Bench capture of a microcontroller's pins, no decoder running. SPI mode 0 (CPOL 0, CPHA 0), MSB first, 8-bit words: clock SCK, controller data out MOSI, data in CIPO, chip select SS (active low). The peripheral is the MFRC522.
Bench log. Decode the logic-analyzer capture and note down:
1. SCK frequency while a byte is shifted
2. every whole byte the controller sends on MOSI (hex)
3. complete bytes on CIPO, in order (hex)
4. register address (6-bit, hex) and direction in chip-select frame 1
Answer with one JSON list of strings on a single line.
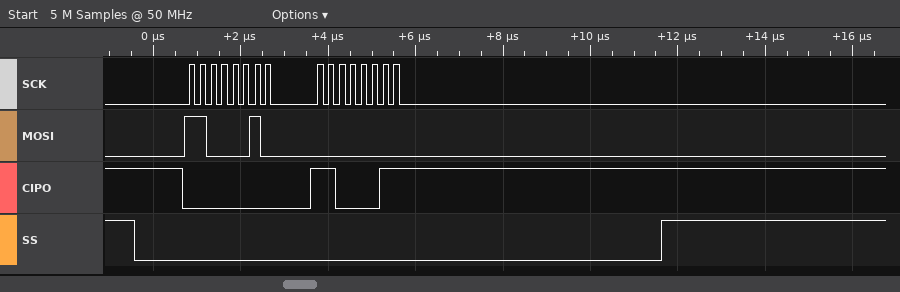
["4 MHz", "C2 00", "00 C3", "0x21 read"]
